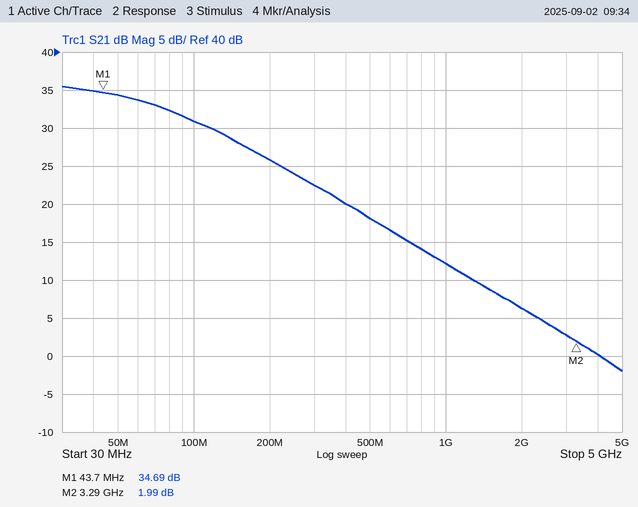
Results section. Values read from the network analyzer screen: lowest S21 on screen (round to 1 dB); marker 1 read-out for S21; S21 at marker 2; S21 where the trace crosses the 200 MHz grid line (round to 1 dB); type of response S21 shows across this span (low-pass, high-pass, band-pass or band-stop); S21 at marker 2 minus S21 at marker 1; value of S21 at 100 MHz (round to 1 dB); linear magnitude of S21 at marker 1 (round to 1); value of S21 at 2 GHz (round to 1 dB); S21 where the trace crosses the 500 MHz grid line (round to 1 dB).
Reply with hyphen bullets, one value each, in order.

- -2 dB
- 34.69 dB
- 1.99 dB
- 26 dB
- low-pass
- -32.70 dB
- 31 dB
- 54
- 6 dB
- 18 dB
